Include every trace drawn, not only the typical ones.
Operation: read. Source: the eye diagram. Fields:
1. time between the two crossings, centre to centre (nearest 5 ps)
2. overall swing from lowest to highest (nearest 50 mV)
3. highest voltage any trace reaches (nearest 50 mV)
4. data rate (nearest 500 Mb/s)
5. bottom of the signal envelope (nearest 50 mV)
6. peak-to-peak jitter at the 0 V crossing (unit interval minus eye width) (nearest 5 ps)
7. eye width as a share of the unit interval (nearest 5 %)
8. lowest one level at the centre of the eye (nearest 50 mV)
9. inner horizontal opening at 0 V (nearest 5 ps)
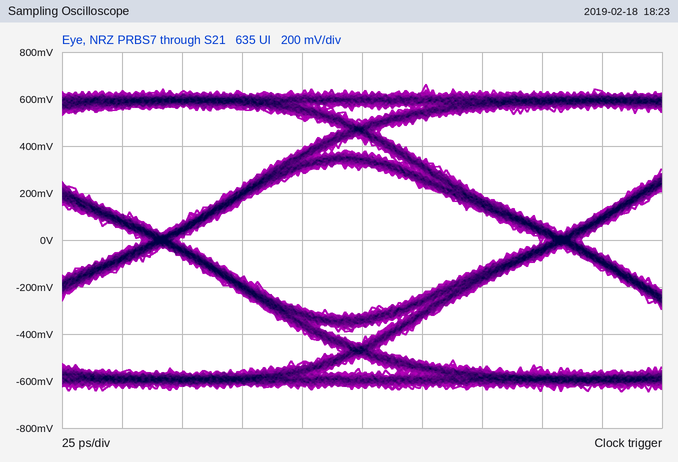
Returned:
165 ps
1.30 V
650 mV
6.0 Gb/s
-650 mV
15 ps
90 %
300 mV
150 ps
